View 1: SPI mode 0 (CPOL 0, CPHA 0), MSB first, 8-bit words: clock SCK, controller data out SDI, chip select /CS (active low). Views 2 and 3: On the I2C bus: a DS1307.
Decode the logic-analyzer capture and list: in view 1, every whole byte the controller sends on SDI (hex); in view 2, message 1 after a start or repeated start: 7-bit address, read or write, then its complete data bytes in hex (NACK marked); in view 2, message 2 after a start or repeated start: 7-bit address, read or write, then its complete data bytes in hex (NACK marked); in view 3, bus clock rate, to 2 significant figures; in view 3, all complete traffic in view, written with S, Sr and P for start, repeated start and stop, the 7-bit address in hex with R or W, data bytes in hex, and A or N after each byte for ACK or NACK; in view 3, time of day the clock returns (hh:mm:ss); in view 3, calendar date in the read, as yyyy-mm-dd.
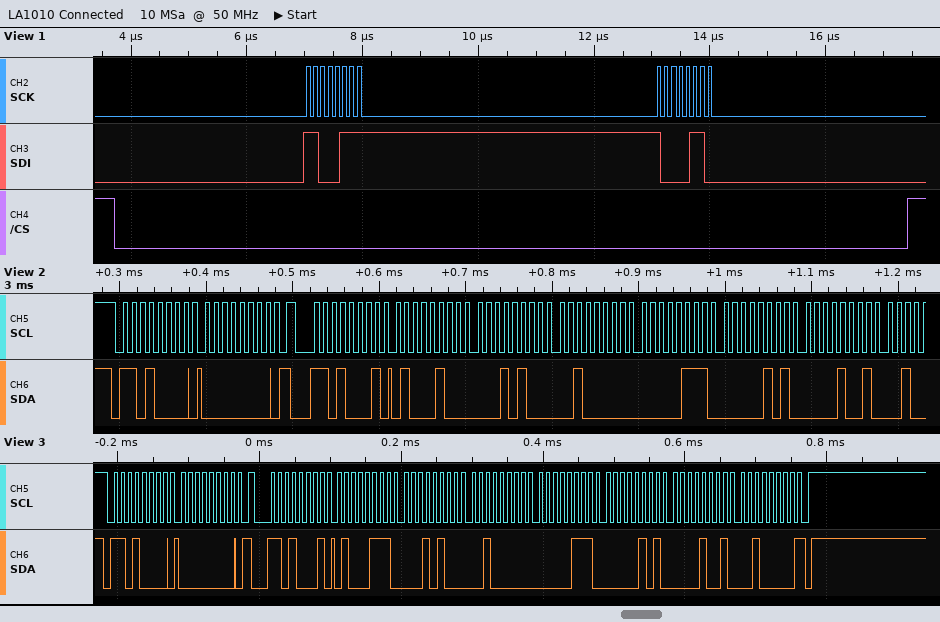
C7 86
0x68 write: 00
0x68 read: 44 14 20 07 05 09
100 kHz
S 68W A 00 A Sr 68R A 47 A 14 A 20 A 07 A 05 A 09 A 20 N P
20:14:47
2020-09-05
